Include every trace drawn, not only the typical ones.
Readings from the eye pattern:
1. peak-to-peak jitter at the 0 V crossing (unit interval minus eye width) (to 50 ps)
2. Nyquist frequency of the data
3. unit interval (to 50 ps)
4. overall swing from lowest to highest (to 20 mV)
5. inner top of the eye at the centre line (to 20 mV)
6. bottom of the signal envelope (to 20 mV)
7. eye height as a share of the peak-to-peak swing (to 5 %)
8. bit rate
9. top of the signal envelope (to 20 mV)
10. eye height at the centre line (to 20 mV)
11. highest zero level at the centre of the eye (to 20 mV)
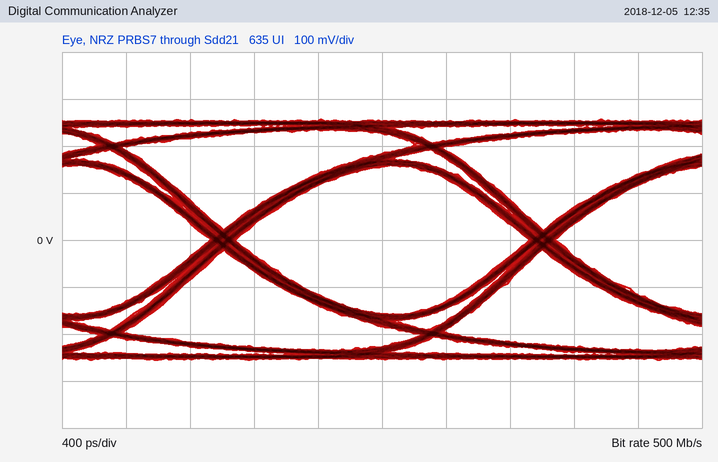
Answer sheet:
150 ps
250 MHz
2.00 ns
520 mV
160 mV
-260 mV
60 %
500 Mb/s
260 mV
320 mV
-160 mV
